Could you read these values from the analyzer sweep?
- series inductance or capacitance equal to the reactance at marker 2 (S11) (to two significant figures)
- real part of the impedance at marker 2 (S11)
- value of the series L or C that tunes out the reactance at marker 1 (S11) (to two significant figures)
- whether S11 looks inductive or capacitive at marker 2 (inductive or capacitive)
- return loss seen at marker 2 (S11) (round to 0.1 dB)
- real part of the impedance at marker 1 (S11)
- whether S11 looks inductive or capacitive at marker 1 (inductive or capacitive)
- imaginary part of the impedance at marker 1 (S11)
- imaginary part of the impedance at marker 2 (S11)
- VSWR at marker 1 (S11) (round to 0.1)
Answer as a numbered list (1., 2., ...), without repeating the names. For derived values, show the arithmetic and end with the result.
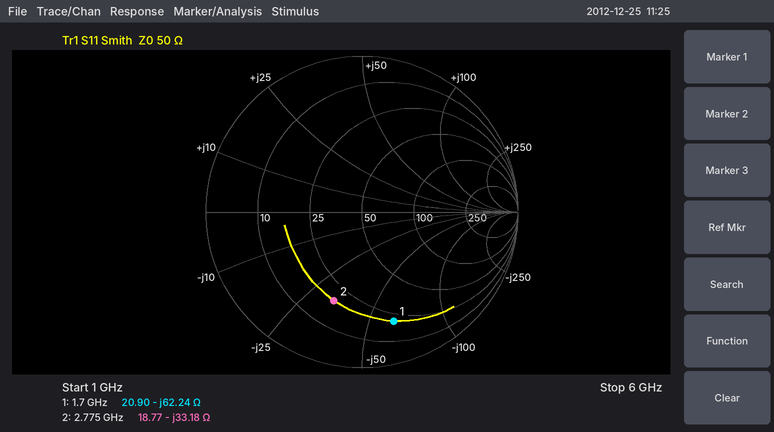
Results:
1. C = 1/(2π × 2.775 GHz × 33.18 Ω) ≈ 1.7 pF
2. 18.77 Ω
3. L = 62.24 Ω/(2π × 1.7 GHz) ≈ 5.8 nH
4. capacitive
5. 4.5 dB
6. 20.90 Ω
7. capacitive
8. -62.24 Ω
9. -33.18 Ω
10. 6.4
